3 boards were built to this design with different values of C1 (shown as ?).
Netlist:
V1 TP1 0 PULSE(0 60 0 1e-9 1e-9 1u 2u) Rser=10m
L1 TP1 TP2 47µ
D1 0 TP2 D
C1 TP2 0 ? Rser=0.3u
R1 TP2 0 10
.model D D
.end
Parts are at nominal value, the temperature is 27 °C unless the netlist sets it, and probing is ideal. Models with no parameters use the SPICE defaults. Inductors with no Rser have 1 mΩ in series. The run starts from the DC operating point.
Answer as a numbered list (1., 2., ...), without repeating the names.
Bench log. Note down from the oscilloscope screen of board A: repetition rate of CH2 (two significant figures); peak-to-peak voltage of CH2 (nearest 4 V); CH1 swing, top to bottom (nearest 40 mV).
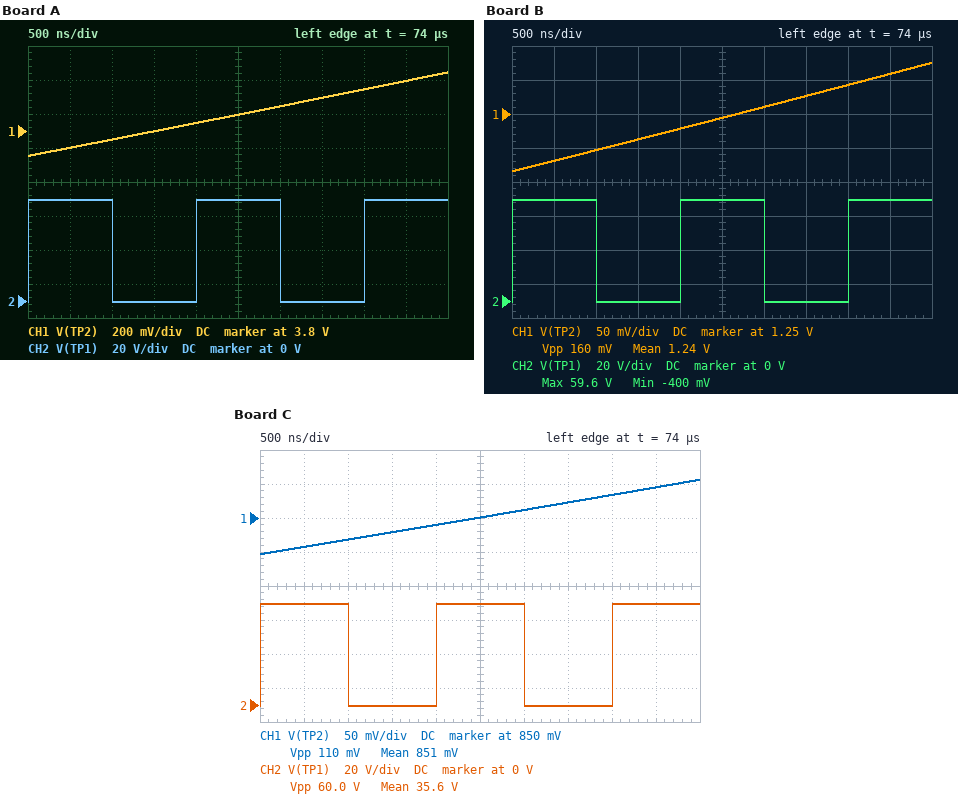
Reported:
1. 500 kHz
2. 60 V
3. 480 mV
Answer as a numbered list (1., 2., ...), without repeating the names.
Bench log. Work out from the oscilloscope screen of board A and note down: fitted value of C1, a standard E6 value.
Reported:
1. 470 µF
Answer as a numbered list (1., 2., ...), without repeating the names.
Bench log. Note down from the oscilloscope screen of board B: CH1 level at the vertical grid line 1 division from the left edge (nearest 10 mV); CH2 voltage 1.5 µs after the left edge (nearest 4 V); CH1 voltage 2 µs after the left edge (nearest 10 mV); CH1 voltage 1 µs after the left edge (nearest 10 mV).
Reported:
1. 1.18 V
2. 0 V
3. 1.23 V
4. 1.20 V
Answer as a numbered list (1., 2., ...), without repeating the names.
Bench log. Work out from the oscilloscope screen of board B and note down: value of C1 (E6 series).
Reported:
1. 1.5 mF
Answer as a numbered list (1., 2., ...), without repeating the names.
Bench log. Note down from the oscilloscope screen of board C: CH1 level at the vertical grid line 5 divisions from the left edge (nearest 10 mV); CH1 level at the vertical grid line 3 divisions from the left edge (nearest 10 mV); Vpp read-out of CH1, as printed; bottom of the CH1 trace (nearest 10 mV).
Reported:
1. 850 mV
2. 830 mV
3. 110 mV
4. 800 mV
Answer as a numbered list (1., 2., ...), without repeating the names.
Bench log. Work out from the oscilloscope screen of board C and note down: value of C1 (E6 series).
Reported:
1. 2.2 mF
